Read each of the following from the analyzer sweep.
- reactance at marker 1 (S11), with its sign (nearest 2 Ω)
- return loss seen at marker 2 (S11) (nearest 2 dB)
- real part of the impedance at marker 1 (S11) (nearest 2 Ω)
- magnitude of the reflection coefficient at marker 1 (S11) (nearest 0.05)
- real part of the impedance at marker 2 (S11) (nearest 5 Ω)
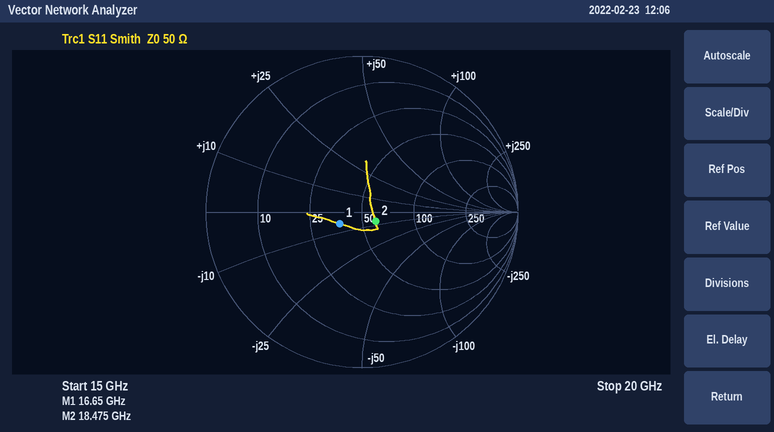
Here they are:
-6 Ω
20 dB
38 Ω
0.15
60 Ω
